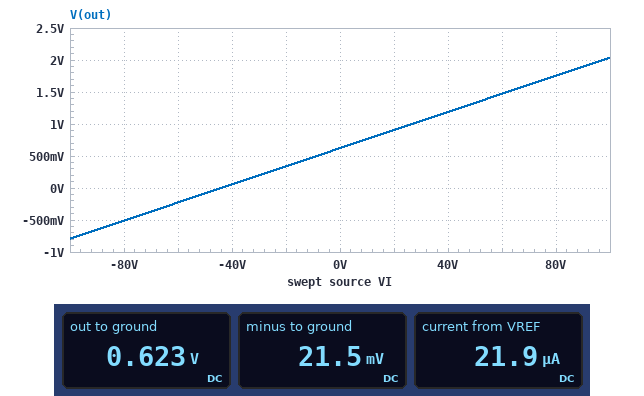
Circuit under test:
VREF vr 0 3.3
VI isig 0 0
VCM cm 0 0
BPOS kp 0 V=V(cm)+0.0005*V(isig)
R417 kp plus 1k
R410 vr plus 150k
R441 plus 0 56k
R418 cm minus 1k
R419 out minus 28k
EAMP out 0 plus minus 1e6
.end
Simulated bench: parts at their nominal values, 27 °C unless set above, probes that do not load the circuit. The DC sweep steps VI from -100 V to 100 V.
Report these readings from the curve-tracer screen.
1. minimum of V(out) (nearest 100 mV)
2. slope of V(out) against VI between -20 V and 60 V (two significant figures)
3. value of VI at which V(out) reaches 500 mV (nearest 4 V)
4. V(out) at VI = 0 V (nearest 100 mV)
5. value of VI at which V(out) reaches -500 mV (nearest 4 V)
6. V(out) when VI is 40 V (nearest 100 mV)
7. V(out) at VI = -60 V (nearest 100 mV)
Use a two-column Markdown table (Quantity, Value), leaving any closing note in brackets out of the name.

| Quantity | Value |
|---|---|
| minimum of V(out) | -800 mV |
| slope of V(out) against VI between -20 V and 60 V | 0.014 V/V |
| value of VI at which V(out) reaches 500 mV | -8 V |
| V(out) at VI = 0 V | 600 mV |
| value of VI at which V(out) reaches -500 mV | -80 V |
| V(out) when VI is 40 V | 1.2 V |
| V(out) at VI = -60 V | -200 mV |
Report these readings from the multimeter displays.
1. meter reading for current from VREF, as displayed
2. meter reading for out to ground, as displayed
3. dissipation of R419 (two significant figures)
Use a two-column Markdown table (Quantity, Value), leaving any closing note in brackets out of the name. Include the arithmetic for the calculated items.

| Quantity | Value |
|---|---|
| meter reading for current from VREF, as displayed | 21.9 µA |
| meter reading for out to ground, as displayed | 0.623 V |
| dissipation of R419 | (623 mV - 21.5 mV)^2 / 28 kΩ = 13 µW |
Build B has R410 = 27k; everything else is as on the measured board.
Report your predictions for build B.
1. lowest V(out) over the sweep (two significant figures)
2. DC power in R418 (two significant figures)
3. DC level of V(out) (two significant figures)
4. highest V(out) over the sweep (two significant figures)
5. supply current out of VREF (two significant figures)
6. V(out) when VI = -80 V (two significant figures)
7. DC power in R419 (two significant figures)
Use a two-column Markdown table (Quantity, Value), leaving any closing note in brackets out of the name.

| Quantity | Value |
|---|---|
| lowest V(out) over the sweep | 2.0 V |
| DC power in R418 | 13 µW |
| DC level of V(out) | 3.4 V |
| highest V(out) over the sweep | 4.7 V |
| supply current out of VREF | 120 µA |
| V(out) when VI = -80 V | 2.3 V |
| DC power in R419 | 380 µW |
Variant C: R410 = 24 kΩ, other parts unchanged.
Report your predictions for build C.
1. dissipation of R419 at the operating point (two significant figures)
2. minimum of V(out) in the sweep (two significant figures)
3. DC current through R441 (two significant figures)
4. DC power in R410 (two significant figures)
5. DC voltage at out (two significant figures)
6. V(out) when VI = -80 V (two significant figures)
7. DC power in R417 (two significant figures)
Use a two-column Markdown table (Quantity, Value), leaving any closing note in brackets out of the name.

| Quantity | Value |
|---|---|
| dissipation of R419 at the operating point | 470 µW |
| minimum of V(out) in the sweep | 2.4 V |
| DC current through R441 | 2.3 µA |
| DC power in R410 | 420 µW |
| DC voltage at out | 3.8 V |
| V(out) when VI = -80 V | 2.7 V |
| DC power in R417 | 17 µW |
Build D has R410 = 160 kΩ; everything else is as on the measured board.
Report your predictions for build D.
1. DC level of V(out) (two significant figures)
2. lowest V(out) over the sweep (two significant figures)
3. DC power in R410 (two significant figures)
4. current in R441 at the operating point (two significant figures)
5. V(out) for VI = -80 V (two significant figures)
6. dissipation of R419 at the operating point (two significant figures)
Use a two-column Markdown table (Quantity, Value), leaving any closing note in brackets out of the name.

| Quantity | Value |
|---|---|
| DC level of V(out) | 580 mV |
| lowest V(out) over the sweep | -830 mV |
| DC power in R410 | 67 µW |
| current in R441 at the operating point | 360 nA |
| V(out) for VI = -80 V | -550 mV |
| dissipation of R419 at the operating point | 11 µW |
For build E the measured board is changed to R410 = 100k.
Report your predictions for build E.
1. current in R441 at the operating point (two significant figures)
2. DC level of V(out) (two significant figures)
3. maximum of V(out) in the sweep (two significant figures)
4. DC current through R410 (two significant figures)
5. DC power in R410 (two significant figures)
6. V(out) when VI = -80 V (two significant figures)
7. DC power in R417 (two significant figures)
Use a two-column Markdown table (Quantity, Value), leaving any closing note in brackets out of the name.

| Quantity | Value |
|---|---|
| current in R441 at the operating point | 570 nA |
| DC level of V(out) | 930 mV |
| maximum of V(out) in the sweep | 2.3 V |
| DC current through R410 | 33 µA |
| DC power in R410 | 110 µW |
| V(out) when VI = -80 V | -200 mV |
| DC power in R417 | 1.0 µW |
